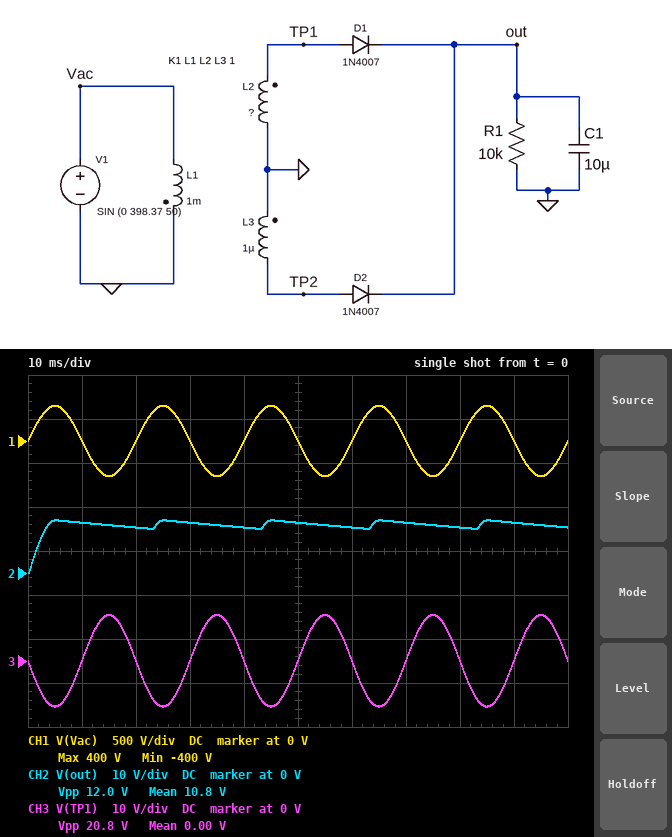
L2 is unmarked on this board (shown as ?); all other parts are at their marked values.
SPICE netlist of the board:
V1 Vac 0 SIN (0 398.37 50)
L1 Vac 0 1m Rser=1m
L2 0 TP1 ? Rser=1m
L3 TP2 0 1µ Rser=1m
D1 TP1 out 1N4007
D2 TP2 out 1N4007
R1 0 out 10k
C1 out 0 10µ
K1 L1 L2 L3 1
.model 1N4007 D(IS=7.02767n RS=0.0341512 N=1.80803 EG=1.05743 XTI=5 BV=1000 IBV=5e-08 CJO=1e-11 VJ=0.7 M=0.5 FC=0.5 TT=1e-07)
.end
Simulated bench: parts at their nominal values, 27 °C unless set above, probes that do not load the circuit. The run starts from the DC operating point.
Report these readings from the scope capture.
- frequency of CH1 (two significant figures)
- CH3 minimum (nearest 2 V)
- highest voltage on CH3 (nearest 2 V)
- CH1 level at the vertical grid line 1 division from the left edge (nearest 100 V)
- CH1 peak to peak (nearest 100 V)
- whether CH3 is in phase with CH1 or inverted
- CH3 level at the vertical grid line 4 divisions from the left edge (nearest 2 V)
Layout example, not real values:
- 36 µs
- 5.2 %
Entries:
- 50 Hz
- -10 V
- 10 V
- 0 V
- 800 V
- inverted
- 0 V
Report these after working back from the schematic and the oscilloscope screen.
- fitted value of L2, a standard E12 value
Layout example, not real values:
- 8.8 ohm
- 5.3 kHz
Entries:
- 680 nH
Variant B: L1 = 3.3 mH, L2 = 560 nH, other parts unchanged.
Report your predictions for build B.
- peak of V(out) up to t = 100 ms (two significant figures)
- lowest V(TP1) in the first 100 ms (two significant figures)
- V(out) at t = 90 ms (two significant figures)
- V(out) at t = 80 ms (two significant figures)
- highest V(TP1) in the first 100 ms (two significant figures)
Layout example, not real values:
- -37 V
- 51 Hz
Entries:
- 6.4 V
- -5.2 V
- 6.1 V
- 5.5 V
- 5.2 V
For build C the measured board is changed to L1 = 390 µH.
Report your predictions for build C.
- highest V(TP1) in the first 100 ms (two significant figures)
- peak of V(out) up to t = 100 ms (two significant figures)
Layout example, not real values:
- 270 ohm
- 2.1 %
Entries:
- 17 V
- 19 V
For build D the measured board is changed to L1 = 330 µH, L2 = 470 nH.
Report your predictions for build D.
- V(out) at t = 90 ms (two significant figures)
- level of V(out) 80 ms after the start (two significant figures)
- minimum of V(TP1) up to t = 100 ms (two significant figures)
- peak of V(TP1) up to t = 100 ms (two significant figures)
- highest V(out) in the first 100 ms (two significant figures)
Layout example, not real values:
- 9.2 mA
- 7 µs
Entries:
- 20 V
- 18 V
- -15 V
- 15 V
- 21 V
